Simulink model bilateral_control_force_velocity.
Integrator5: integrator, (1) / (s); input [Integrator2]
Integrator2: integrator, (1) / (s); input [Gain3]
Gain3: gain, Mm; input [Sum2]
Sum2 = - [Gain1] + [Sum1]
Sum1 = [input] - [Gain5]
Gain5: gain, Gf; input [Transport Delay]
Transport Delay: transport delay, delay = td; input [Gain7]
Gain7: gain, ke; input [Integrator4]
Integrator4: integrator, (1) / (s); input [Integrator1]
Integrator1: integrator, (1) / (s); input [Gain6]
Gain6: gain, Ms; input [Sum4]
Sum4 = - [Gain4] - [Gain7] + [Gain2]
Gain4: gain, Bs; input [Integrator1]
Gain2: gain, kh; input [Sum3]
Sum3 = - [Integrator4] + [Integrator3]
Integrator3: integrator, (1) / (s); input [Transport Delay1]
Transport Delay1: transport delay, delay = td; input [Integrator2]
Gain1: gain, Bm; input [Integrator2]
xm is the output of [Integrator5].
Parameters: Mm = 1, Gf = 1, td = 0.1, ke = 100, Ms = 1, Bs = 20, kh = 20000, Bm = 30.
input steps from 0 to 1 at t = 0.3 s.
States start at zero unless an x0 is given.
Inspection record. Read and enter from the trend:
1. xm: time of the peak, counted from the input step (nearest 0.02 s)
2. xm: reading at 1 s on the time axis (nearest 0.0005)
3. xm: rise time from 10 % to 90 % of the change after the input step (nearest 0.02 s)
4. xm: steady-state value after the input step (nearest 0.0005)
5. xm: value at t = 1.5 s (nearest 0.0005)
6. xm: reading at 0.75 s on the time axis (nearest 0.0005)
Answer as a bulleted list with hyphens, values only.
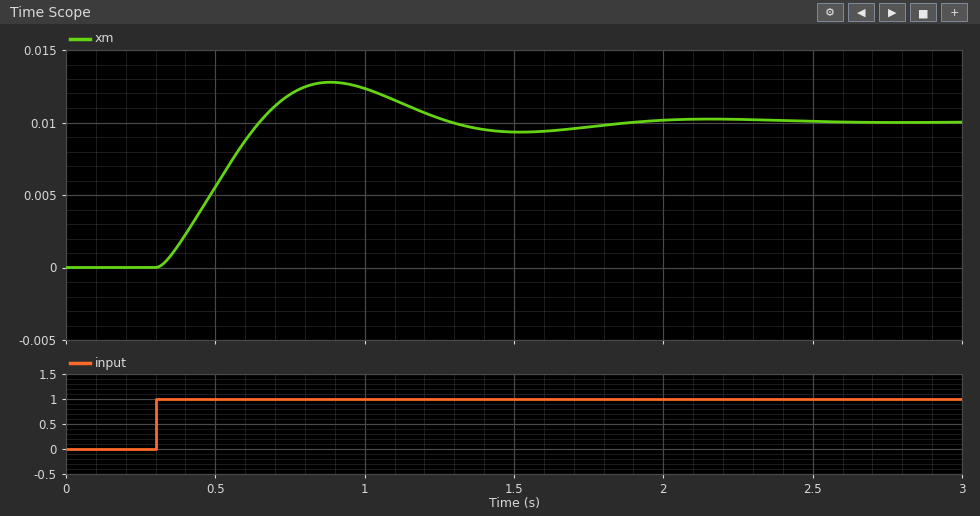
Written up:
- 0.58 s
- 0.0125
- 0.26 s
- 0.0100
- 0.0095
- 0.0120
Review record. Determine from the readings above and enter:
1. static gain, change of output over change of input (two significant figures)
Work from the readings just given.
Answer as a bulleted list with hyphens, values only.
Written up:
- 0.010
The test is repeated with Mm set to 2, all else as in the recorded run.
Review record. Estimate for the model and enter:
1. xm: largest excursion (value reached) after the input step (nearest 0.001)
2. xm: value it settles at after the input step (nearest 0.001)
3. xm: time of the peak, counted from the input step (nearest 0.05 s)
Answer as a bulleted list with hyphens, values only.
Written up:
- 0.012
- 0.010
- 0.55 s
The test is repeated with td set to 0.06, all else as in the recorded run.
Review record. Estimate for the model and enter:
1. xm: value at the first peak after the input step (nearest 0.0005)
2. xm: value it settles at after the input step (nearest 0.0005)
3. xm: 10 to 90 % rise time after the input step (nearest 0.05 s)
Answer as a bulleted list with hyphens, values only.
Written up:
- 0.0105
- 0.0100
- 0.30 s
